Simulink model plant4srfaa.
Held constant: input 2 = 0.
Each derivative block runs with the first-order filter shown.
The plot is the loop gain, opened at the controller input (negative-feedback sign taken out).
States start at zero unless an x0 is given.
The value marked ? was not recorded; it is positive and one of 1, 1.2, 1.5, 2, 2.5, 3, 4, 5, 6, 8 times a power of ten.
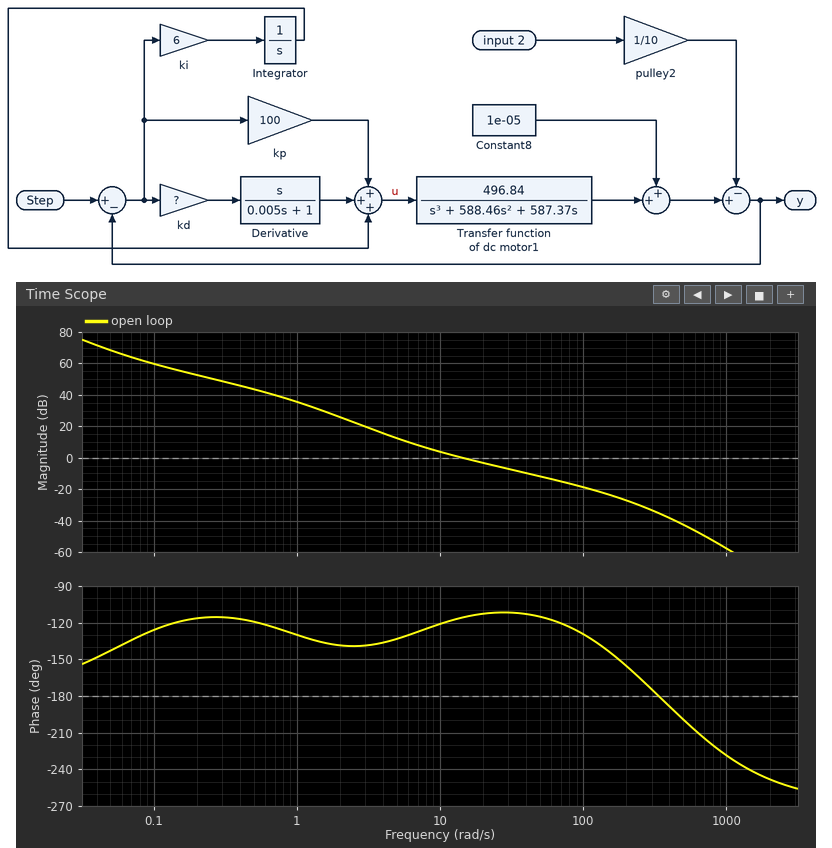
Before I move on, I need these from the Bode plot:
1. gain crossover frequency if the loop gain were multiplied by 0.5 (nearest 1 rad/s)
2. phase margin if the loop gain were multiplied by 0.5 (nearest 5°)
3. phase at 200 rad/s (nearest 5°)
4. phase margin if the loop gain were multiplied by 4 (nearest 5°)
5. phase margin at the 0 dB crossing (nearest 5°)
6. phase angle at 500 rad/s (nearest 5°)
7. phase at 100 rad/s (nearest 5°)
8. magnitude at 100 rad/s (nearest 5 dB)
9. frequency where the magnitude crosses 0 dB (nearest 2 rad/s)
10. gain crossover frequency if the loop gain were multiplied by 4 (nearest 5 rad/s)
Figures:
8 rad/s
55°
-155°
65°
65°
-200°
-130°
-20 dB
14 rad/s
50 rad/s
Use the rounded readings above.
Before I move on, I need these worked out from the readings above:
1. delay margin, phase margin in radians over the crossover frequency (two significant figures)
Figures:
0.081 s
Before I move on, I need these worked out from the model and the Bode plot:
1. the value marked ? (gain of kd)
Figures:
15
